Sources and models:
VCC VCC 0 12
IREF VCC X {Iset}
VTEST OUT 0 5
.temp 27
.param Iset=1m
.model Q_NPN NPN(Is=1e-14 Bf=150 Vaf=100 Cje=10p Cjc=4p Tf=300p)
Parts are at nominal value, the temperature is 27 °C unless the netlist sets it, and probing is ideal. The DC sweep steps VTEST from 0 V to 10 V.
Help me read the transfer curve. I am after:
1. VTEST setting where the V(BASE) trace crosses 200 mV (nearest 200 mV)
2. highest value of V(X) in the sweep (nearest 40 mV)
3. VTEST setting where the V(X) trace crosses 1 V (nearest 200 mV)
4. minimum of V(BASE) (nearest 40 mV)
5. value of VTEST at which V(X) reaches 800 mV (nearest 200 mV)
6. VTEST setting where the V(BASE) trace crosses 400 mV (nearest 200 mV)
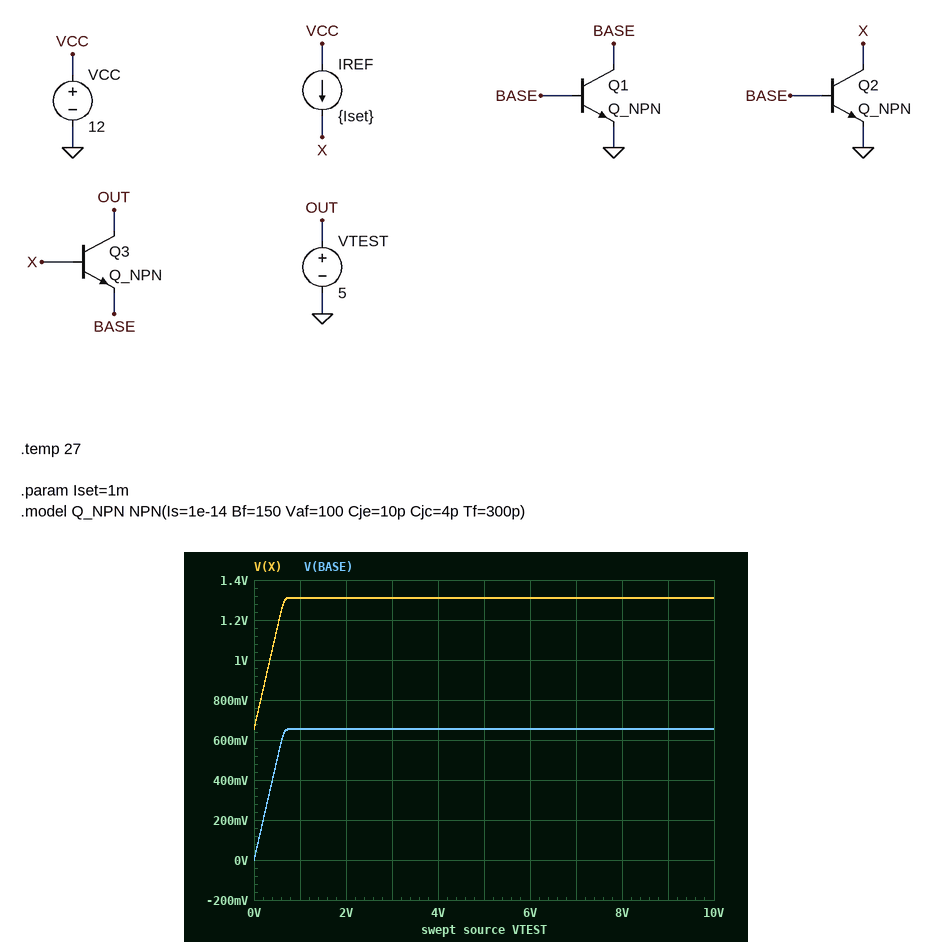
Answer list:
200 mV
1.32 V
400 mV
0 V
200 mV
400 mV
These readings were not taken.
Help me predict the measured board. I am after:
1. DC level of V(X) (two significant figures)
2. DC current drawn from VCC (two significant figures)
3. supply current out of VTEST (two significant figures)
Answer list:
1.3 V
1.0 mA
990 µA
